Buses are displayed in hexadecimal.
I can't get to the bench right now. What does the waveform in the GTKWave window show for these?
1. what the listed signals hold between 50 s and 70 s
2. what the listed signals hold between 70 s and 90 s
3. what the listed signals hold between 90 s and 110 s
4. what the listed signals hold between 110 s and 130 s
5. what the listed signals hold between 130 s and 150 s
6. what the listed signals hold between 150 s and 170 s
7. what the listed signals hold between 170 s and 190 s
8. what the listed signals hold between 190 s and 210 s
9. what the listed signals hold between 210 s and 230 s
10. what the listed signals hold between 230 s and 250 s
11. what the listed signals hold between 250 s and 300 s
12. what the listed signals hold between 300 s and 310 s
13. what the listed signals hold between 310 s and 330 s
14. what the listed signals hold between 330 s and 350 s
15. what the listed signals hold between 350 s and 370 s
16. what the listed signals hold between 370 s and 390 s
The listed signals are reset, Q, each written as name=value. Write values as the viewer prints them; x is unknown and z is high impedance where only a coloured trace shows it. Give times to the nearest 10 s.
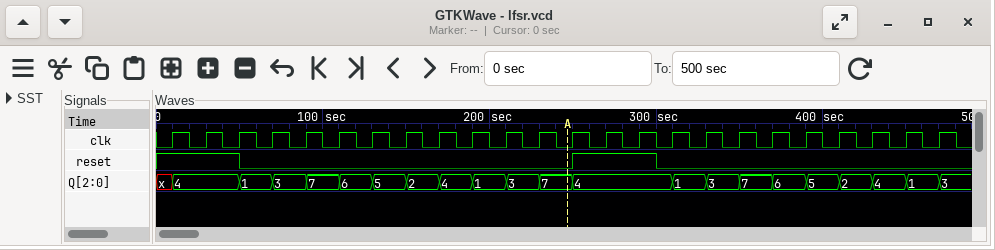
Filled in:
reset=0, Q=1
reset=0, Q=3
reset=0, Q=7
reset=0, Q=6
reset=0, Q=5
reset=0, Q=2
reset=0, Q=4
reset=0, Q=1
reset=0, Q=3
reset=0, Q=7
reset=1, Q=4
reset=0, Q=4
reset=0, Q=1
reset=0, Q=3
reset=0, Q=7
reset=0, Q=6
